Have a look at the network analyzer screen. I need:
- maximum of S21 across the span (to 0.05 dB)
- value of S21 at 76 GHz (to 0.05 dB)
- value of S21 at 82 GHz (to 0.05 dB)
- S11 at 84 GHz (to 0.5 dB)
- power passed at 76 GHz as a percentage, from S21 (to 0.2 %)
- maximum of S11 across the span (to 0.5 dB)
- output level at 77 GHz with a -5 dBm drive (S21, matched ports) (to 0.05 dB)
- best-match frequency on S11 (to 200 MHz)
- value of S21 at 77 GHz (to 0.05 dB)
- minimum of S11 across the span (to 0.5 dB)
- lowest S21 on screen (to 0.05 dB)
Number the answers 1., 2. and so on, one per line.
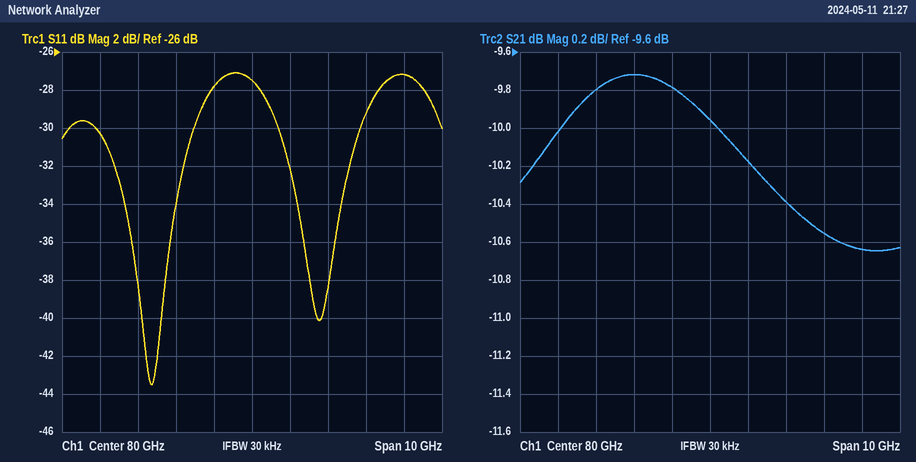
1. -9.70 dB
2. -10.00 dB
3. -10.40 dB
4. -27.0 dB
5. 10.0 %
6. -27.0 dB
7. -14.80 dBm
8. 77.4 GHz
9. -9.80 dB
10. -43.5 dB
11. -10.65 dB
